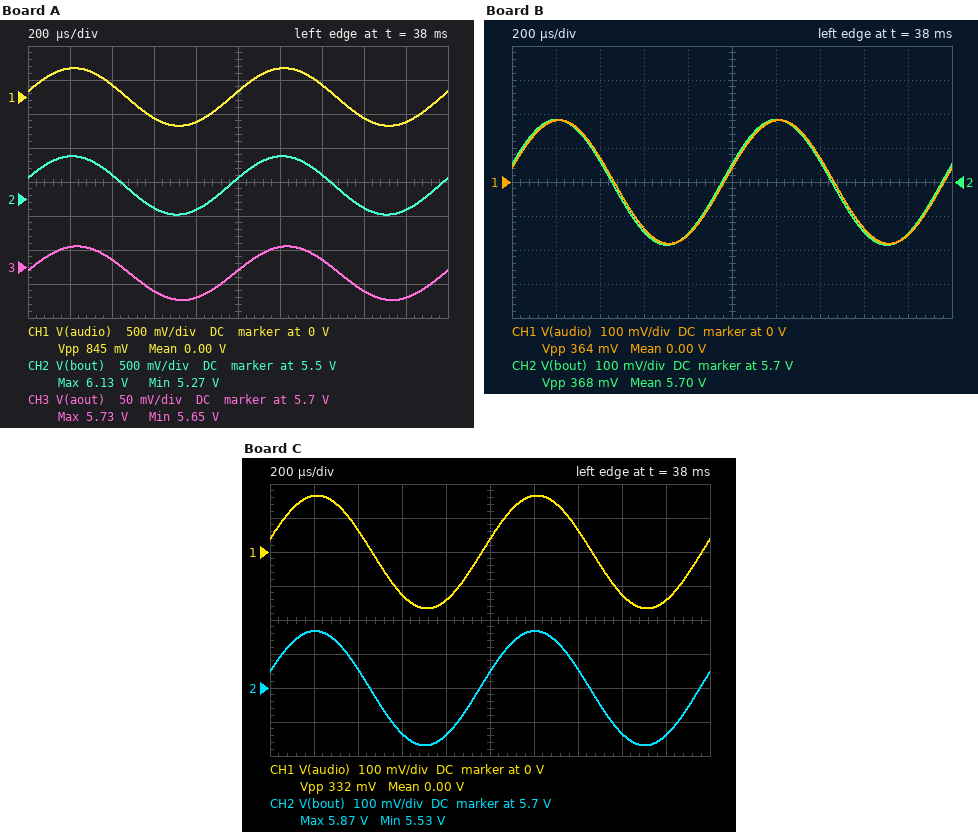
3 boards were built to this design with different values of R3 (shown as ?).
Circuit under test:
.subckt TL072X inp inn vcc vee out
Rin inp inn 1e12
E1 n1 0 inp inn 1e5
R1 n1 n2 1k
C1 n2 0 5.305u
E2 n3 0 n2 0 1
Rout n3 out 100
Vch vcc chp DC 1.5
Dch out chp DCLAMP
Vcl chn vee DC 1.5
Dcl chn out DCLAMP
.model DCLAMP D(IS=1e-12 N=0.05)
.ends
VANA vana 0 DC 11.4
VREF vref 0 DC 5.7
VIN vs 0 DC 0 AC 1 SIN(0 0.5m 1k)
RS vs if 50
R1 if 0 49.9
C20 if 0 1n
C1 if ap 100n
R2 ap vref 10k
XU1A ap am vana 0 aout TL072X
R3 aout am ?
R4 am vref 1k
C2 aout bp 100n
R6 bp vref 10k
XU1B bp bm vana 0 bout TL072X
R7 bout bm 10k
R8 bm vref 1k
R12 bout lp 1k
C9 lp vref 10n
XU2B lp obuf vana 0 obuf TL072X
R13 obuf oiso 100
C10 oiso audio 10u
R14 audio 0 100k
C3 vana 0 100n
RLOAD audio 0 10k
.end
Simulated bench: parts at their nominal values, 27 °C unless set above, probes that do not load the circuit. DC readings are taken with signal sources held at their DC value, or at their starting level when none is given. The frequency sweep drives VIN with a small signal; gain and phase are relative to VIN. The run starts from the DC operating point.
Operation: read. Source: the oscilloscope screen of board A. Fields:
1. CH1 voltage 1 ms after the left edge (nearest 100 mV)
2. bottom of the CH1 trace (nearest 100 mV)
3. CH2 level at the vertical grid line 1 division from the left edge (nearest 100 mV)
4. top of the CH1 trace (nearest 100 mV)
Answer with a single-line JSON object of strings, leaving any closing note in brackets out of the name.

{"CH1 voltage 1 ms after the left edge": "100 mV", "bottom of the CH1 trace": "-400 mV", "CH2 level at the vertical grid line 1 division from the left edge": "6.1 V", "top of the CH1 trace": "400 mV"}
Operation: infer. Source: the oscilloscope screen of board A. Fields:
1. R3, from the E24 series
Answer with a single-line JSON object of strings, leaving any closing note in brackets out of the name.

{"R3, from the E24 series": "160 kΩ"}
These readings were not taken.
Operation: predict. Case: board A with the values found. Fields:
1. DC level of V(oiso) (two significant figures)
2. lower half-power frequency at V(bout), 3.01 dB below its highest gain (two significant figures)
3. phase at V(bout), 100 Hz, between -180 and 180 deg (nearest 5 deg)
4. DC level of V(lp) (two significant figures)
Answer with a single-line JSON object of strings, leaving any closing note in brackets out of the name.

{"DC level of V(oiso)": "5.7 V", "lower half-power frequency at V(bout), 3.01 dB below its highest gain": "240 Hz", "phase at V(bout), 100 Hz, between -180 and 180 deg": "115 deg", "DC level of V(lp)": "5.7 V"}
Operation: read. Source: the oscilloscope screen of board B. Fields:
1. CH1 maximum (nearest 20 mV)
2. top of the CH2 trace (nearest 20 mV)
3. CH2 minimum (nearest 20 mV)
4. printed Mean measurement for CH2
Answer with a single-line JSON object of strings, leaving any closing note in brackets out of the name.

{"CH1 maximum": "180 mV", "top of the CH2 trace": "5.88 V", "CH2 minimum": "5.52 V", "printed Mean measurement for CH2": "5.70 V"}
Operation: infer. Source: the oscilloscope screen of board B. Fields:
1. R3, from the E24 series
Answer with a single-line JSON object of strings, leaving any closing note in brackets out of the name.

{"R3, from the E24 series": "68 kΩ"}
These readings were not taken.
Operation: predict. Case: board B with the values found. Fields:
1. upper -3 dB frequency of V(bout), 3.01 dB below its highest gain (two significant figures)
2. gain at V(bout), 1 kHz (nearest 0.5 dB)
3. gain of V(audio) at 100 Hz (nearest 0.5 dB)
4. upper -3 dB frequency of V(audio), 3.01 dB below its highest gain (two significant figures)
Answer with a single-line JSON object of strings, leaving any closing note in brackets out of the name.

{"upper -3 dB frequency of V(bout), 3.01 dB below its highest gain": "43 kHz", "gain at V(bout), 1 kHz": "51.5 dB", "gain of V(audio) at 100 Hz": "40.5 dB", "upper -3 dB frequency of V(audio), 3.01 dB below its highest gain": "15 kHz"}
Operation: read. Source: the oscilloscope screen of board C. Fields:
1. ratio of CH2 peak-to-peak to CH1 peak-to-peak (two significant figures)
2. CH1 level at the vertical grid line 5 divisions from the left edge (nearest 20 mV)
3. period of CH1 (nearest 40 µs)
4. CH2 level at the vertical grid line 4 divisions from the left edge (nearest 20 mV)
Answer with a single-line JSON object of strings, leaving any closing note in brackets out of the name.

{"ratio of CH2 peak-to-peak to CH1 peak-to-peak": "1.0", "CH1 level at the vertical grid line 5 divisions from the left edge": "40 mV", "period of CH1": "1.00 ms", "CH2 level at the vertical grid line 4 divisions from the left edge": "5.56 V"}
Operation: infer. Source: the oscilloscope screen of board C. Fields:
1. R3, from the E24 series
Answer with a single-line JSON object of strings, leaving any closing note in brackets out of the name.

{"R3, from the E24 series": "62 kΩ"}
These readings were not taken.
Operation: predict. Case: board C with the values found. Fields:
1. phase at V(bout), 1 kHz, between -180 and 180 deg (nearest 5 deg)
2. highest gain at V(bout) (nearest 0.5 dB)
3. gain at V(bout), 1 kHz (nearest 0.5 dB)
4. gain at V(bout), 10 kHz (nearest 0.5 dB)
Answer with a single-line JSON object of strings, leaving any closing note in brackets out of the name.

{"phase at V(bout), 1 kHz, between -180 and 180 deg": "15 deg", "highest gain at V(bout)": "50.5 dB", "gain at V(bout), 1 kHz": "50.5 dB", "gain at V(bout), 10 kHz": "50.5 dB"}
